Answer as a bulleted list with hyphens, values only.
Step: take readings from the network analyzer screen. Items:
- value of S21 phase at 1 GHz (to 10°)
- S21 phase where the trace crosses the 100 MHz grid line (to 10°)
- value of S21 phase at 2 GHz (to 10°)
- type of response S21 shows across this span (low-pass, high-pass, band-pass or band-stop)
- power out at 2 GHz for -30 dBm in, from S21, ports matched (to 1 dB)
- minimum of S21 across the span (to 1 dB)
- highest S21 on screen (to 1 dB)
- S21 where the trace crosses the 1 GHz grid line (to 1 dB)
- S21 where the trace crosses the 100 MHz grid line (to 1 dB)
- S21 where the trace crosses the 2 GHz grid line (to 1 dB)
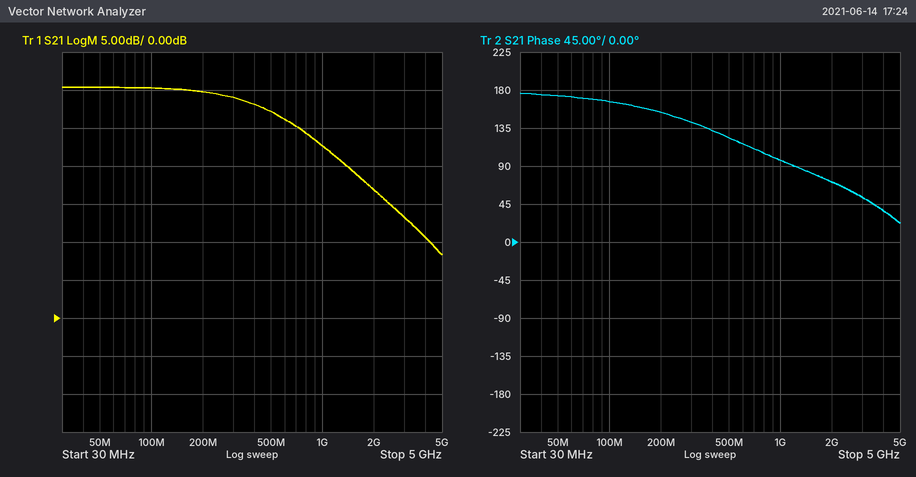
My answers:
- 100°
- 170°
- 70°
- low-pass
- -13 dBm
- 8 dB
- 30 dB
- 23 dB
- 30 dB
- 17 dB
